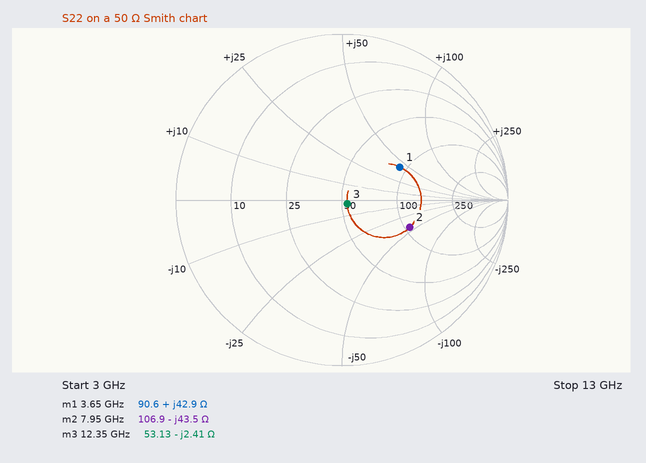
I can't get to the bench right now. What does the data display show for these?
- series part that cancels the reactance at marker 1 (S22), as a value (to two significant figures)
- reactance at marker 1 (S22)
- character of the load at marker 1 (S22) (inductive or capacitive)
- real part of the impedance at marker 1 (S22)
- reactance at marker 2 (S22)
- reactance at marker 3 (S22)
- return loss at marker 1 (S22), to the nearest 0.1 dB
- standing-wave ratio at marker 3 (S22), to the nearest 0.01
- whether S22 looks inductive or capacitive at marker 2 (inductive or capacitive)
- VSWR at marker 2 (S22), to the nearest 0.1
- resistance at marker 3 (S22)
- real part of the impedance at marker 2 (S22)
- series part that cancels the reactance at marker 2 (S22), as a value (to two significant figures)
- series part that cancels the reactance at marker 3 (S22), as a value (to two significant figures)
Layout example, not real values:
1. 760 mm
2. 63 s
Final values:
1. 1.0 pF
2. +42.9 Ω
3. inductive
4. 90.6 Ω
5. -43.5 Ω
6. -2.41 Ω
7. 7.9 dB
8. 1.08
9. capacitive
10. 2.6
11. 53.13 Ω
12. 106.9 Ω
13. 870 pH
14. 31 pH
